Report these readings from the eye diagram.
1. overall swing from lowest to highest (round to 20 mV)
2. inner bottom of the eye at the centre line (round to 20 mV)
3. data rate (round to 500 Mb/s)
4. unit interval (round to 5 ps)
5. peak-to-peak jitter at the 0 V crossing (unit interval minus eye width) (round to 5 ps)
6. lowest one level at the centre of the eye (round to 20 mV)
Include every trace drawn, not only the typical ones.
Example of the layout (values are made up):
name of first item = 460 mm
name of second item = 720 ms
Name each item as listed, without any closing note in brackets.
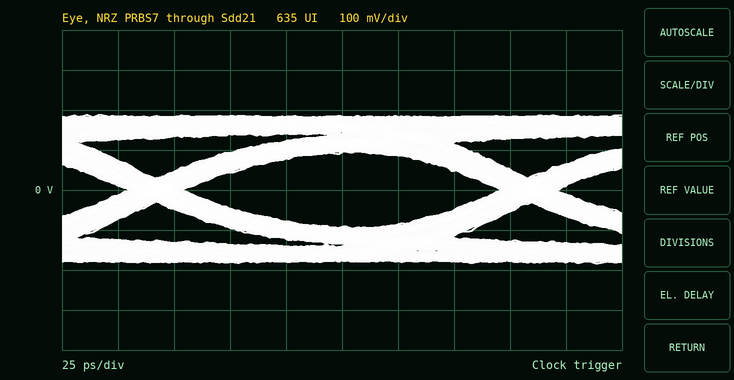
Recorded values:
overall swing from lowest to highest = 380 mV
inner bottom of the eye at the centre line = -100 mV
data rate = 6.0 Gb/s
unit interval = 165 ps
peak-to-peak jitter at the 0 V crossing (unit interval minus eye width) = 25 ps
lowest one level at the centre of the eye = 100 mV
